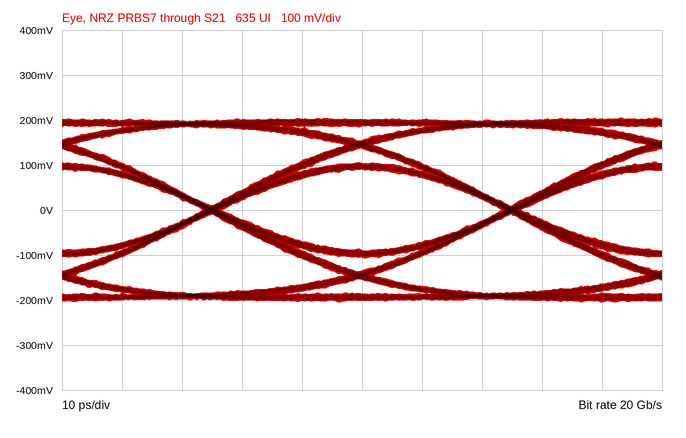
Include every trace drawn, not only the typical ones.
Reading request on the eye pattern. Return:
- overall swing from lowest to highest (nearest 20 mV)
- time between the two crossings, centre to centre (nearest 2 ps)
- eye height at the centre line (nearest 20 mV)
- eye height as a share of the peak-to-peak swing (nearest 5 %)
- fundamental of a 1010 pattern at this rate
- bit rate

400 mV
50 ps
180 mV
45 %
10 GHz
20 Gb/s
